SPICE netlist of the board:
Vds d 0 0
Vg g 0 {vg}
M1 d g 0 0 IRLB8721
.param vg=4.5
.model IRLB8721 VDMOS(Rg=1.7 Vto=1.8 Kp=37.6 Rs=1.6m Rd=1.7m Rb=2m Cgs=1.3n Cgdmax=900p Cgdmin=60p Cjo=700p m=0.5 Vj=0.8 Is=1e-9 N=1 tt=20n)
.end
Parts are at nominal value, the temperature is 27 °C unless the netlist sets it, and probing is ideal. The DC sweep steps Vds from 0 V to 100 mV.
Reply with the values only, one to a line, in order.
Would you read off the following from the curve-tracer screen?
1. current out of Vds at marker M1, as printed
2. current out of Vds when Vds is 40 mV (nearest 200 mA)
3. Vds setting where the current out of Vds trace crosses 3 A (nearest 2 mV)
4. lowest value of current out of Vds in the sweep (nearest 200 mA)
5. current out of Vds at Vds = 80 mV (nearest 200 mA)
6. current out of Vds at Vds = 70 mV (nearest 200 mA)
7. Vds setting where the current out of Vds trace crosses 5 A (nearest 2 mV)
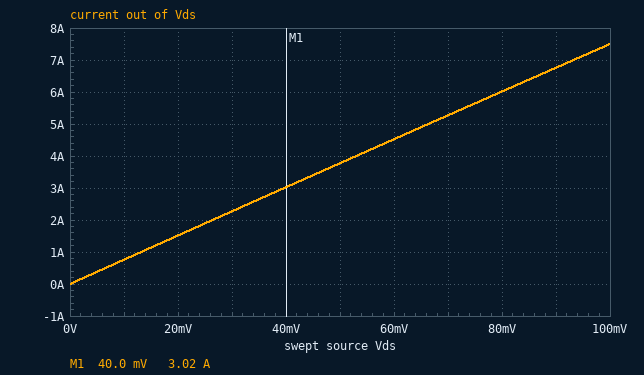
3.02 A
3.0 A
40 mV
0 A
6.0 A
5.2 A
66 mV
